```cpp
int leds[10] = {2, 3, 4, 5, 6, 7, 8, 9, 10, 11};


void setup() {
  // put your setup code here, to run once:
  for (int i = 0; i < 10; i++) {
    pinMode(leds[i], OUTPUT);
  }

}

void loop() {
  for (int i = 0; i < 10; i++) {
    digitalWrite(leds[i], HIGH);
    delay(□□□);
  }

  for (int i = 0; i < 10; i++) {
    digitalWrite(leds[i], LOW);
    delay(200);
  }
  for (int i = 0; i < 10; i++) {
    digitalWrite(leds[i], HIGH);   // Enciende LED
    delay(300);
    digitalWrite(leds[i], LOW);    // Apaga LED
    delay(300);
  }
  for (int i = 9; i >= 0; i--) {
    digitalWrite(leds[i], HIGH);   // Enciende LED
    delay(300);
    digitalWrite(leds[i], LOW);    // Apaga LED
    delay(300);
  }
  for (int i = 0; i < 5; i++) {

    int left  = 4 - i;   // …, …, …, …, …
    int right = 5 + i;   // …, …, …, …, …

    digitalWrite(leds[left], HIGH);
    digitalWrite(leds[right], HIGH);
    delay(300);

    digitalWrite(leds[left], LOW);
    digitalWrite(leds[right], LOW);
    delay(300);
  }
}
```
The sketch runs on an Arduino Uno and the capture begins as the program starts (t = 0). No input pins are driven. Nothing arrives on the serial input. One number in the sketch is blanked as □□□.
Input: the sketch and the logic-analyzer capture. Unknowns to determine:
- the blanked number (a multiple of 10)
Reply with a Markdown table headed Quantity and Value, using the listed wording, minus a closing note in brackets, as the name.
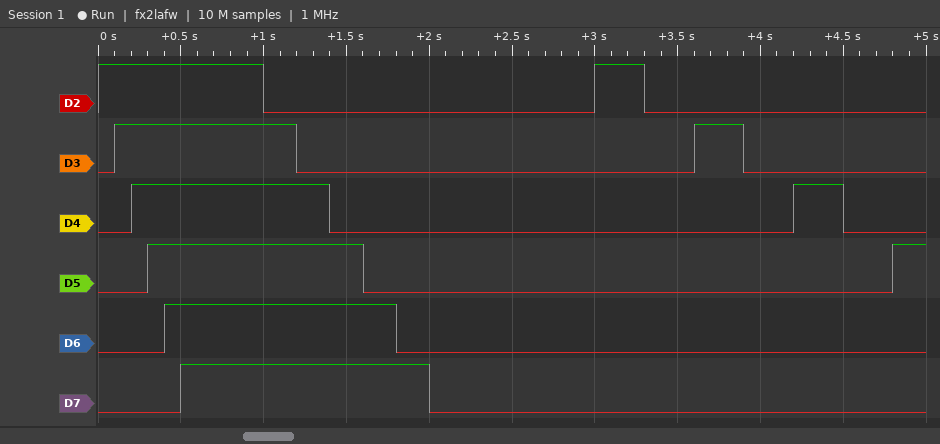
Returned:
| Quantity | Value |
|---|---|
| the blanked number | 100 |
